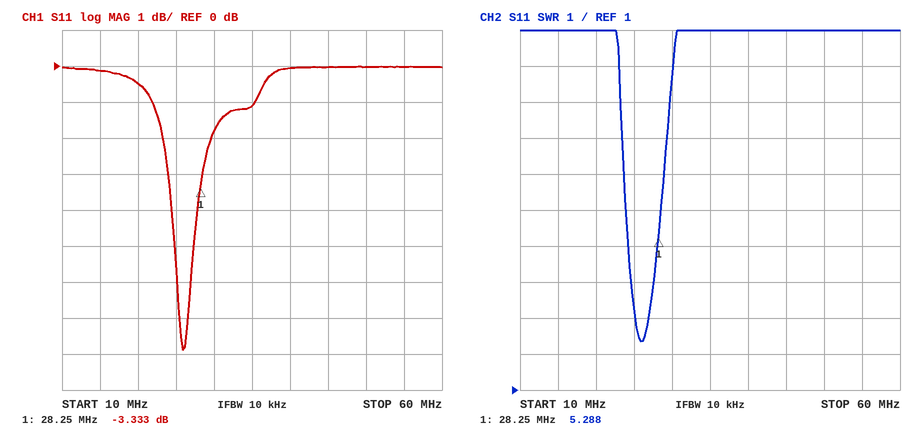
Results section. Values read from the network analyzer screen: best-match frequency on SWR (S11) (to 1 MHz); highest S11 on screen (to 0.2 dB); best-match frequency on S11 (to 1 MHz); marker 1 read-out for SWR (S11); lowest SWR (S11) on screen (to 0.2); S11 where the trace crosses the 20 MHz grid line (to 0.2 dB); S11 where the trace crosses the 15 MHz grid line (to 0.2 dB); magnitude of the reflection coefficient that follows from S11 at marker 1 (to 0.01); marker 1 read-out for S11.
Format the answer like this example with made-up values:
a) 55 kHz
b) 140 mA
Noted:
a) 26 MHz
b) 0.0 dB
c) 26 MHz
d) 5.288
e) 2.4
f) -0.4 dB
g) -0.2 dB
h) 0.68
i) -3.333 dB
